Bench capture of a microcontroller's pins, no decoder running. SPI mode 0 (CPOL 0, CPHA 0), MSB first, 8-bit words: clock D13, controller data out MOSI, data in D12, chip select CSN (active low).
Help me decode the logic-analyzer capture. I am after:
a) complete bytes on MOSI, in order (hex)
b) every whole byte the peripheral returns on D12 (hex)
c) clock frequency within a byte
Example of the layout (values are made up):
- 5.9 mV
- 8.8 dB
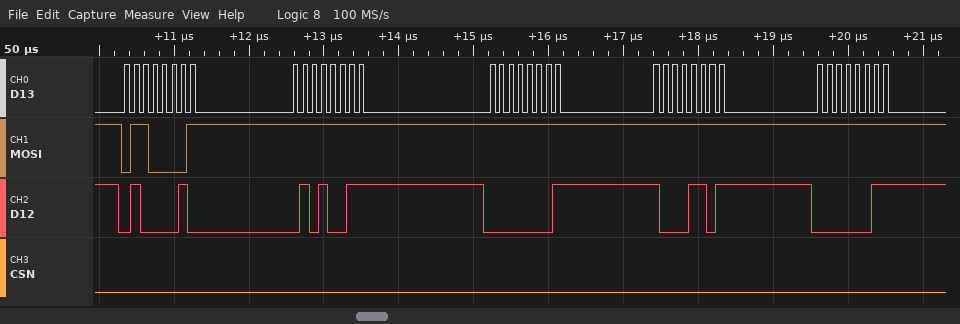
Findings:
- 61 FF FF FF FF
- 42 53 01 8D 03
- 8 MHz
